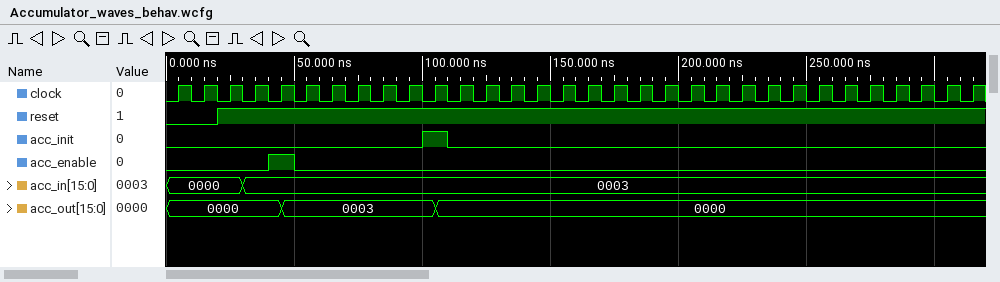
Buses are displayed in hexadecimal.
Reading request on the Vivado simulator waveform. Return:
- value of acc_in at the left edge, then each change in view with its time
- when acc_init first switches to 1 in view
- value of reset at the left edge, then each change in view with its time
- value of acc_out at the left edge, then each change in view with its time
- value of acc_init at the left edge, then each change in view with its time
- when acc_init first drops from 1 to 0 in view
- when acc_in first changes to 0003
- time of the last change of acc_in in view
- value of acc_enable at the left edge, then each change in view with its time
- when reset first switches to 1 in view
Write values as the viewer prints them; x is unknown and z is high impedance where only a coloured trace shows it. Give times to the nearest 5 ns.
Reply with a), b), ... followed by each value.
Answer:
a) 0000, 0003 at 30 ns
b) 100 ns
c) 0, 1 at 20 ns
d) 0000, 0003 at 45 ns, 0000 at 105 ns
e) 0, 1 at 100 ns, 0 at 110 ns
f) 110 ns
g) 30 ns
h) 30 ns
i) 0, 1 at 40 ns, 0 at 50 ns
j) 20 ns
